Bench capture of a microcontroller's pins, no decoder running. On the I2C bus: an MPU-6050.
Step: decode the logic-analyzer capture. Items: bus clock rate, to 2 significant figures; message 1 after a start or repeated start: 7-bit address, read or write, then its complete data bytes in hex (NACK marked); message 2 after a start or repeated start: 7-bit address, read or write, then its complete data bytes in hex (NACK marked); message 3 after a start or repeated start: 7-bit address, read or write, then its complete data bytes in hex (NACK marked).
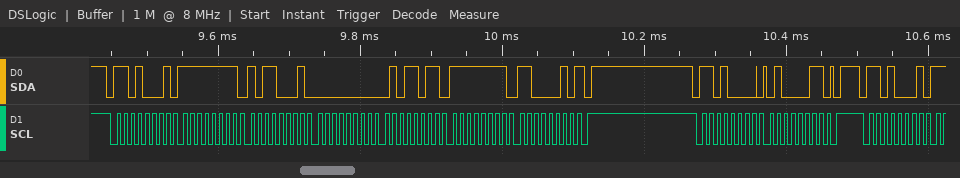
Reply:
100 kHz
0x68 read: FF B1 00 5B FF C2 NACK
0x68 write: 43
0x68 read
